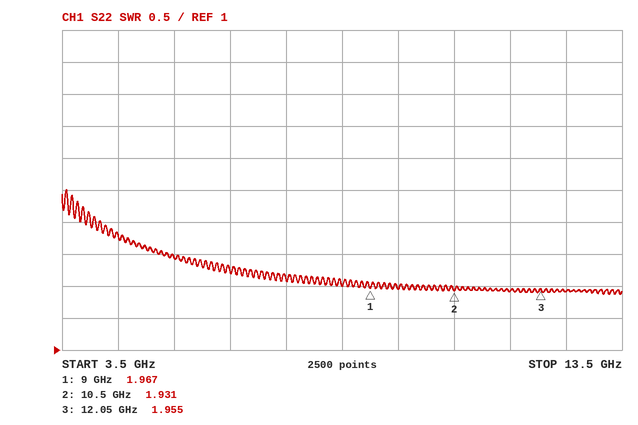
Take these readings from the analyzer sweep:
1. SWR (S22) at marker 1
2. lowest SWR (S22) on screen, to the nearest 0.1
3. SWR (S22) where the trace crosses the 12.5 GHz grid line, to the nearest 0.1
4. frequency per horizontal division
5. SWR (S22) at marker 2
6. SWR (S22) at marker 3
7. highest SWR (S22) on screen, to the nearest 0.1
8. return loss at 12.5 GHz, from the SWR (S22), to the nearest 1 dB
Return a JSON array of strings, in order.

["1.967", "1.9", "1.9", "1 GHz", "1.931", "1.955", "3.5", "10 dB"]
